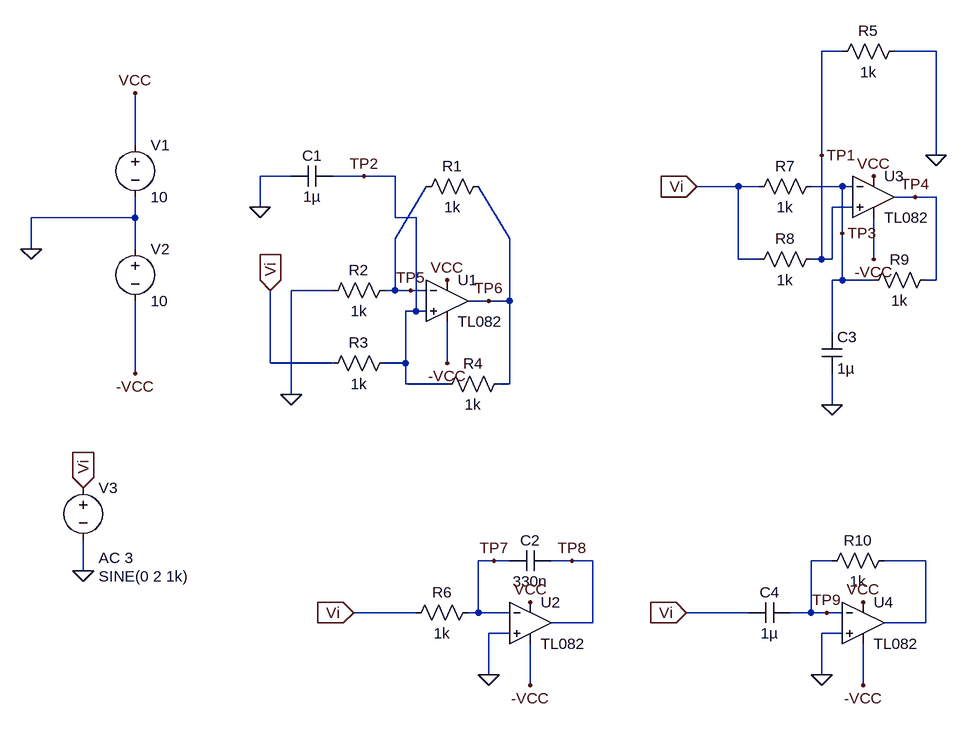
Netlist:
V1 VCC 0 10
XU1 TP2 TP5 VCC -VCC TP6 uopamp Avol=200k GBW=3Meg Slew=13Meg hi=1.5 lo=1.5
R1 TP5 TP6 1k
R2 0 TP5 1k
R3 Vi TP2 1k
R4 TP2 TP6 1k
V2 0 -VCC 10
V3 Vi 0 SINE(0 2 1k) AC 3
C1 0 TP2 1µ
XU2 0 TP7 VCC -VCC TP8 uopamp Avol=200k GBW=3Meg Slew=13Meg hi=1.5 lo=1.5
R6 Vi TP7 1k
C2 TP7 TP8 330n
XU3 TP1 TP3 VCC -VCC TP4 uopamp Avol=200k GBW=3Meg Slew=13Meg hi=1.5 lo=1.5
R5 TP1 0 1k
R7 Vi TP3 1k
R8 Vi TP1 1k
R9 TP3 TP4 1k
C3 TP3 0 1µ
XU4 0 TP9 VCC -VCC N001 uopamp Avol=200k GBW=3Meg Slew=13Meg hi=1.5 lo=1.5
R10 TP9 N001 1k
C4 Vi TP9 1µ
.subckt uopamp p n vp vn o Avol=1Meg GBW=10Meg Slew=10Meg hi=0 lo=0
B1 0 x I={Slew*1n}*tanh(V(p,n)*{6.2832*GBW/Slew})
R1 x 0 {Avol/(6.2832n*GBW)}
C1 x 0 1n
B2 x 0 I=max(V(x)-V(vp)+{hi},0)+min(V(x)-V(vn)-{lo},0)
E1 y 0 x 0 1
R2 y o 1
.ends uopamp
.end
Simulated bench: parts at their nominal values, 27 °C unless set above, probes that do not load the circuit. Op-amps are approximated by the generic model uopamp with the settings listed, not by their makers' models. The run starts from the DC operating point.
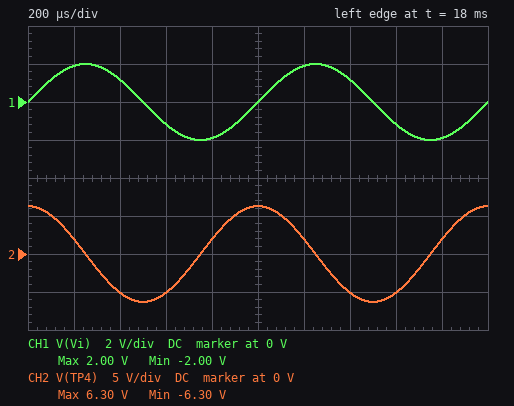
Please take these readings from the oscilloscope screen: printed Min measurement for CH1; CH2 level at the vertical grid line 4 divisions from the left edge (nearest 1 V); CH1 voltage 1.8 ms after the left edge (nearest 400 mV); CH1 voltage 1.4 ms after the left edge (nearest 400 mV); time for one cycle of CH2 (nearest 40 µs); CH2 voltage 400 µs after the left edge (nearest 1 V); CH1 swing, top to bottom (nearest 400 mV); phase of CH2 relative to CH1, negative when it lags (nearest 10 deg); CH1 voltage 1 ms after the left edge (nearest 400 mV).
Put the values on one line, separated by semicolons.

-2.00 V; 2 V; -2.0 V; 1.2 V; 1.00 ms; -5 V; 4.0 V; 90 deg; 0 V
